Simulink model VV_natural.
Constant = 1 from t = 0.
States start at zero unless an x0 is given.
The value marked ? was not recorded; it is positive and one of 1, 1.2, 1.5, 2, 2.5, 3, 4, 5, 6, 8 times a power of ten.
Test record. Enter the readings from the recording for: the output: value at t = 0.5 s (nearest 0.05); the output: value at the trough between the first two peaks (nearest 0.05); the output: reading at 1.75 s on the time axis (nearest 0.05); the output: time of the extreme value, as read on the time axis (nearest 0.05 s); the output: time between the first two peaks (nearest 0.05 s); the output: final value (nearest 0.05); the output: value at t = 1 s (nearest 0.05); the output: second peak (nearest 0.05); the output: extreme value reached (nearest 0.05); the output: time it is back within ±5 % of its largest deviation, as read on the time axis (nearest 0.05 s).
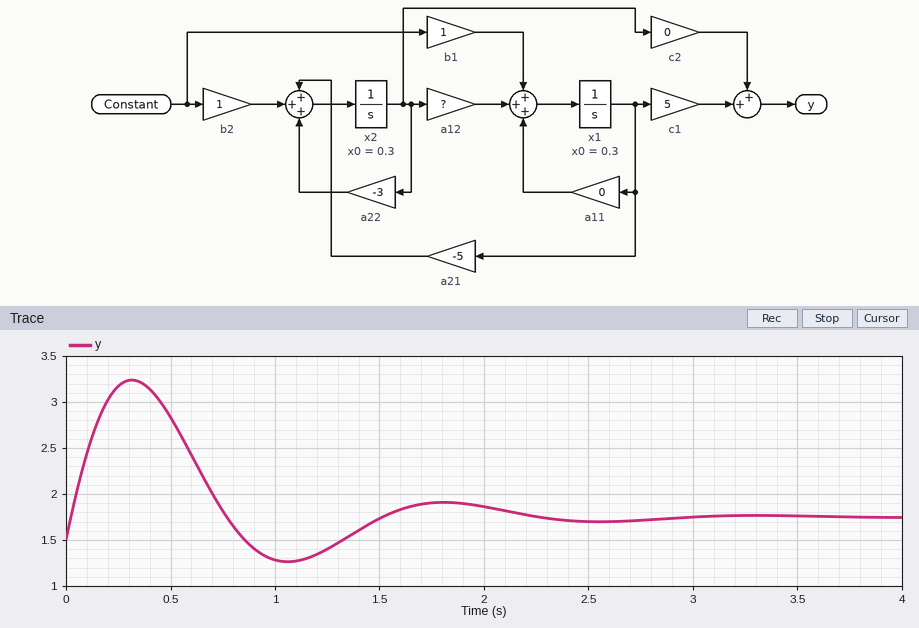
2.85
1.25
1.90
0.30 s
1.50 s
1.75
1.30
1.90
3.25
2.05 s
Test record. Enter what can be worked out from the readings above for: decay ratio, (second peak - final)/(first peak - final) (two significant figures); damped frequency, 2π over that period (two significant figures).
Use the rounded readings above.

0.10
4.2 rad/s
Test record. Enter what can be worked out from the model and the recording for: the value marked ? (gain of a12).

4
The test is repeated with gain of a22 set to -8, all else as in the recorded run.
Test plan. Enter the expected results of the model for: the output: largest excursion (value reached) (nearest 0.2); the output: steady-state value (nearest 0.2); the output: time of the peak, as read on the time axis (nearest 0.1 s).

3.2
3.0
0.5 s
